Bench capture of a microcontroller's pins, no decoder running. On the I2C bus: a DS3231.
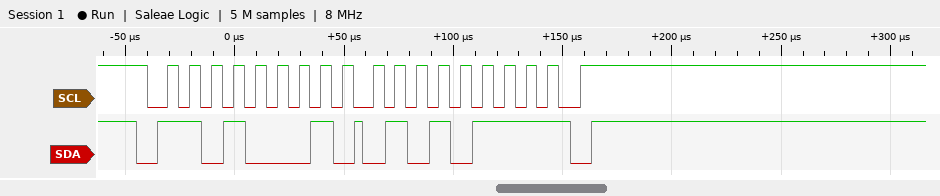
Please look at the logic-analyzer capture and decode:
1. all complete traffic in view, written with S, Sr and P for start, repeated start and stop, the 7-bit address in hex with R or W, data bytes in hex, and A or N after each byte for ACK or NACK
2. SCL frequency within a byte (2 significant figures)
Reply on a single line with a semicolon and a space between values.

S 68R A 57 N P; 100 kHz
